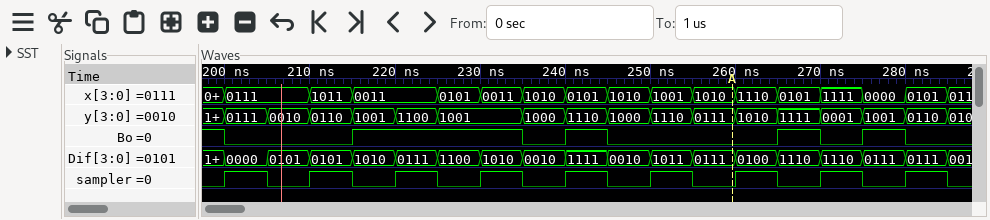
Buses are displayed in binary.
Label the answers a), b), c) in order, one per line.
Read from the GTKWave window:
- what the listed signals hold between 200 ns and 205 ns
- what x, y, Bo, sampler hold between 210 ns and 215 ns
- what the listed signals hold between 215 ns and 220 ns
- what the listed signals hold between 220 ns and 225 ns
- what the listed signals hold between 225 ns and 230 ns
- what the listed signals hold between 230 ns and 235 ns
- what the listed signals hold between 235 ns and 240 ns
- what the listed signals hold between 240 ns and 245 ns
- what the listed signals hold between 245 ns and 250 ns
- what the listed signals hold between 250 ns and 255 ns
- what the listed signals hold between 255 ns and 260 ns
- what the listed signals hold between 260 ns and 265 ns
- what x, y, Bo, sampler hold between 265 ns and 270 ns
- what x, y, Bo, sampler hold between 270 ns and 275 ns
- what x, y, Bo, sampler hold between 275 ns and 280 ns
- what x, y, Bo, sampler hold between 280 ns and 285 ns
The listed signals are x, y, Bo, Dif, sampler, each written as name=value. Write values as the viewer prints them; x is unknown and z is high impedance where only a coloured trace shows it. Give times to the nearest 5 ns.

a) x=0111, y=0111, Bo=0, Dif=0000, sampler=1
b) x=1011, y=0110, Bo=0, sampler=1
c) x=0011, y=1001, Bo=1, Dif=1010, sampler=0
d) x=0011, y=1100, Bo=1, Dif=0111, sampler=1
e) x=0101, y=1001, Bo=1, Dif=1100, sampler=0
f) x=0011, y=1001, Bo=1, Dif=1010, sampler=1
g) x=1010, y=1000, Bo=0, Dif=0010, sampler=0
h) x=0101, y=1110, Bo=1, Dif=1111, sampler=1
i) x=1010, y=1000, Bo=0, Dif=0010, sampler=0
j) x=1001, y=1110, Bo=0, Dif=1011, sampler=1
k) x=1010, y=0111, Bo=0, Dif=0111, sampler=0
l) x=1110, y=1010, Bo=0, Dif=0100, sampler=1
m) x=0101, y=1111, Bo=1, sampler=0
n) x=1111, y=0001, Bo=0, sampler=1
o) x=0000, y=1001, Bo=1, sampler=0
p) x=0101, y=0110, Bo=0, sampler=1
